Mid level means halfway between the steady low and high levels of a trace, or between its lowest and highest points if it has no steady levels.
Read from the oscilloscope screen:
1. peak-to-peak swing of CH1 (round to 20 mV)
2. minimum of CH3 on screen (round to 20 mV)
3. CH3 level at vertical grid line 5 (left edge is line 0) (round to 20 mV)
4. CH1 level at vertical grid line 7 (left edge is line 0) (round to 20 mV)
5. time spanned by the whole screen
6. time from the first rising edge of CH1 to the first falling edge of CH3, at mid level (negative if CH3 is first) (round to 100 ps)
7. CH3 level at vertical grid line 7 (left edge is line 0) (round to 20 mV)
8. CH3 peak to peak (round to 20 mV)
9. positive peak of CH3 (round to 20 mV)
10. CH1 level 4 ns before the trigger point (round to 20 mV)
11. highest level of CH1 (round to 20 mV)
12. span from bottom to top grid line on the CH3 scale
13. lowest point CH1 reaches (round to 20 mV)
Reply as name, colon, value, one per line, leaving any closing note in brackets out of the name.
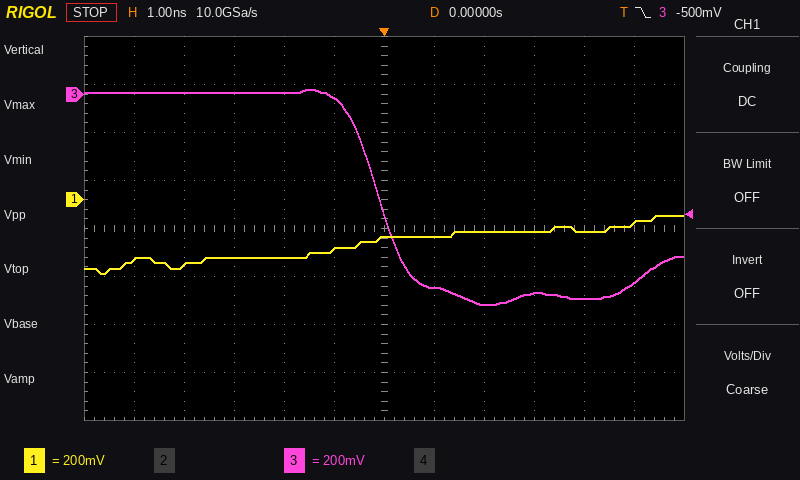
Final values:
peak-to-peak swing of CH1: 240 mV
minimum of CH3 on screen: -880 mV
CH3 level at vertical grid line 5 (left edge is line 0): -20 mV
CH1 level at vertical grid line 7 (left edge is line 0): -160 mV
time spanned by the whole screen: 12 ns
time from the first rising edge of CH1 to the first falling edge of CH3, at mid level (negative if CH3 is first): +400 ps
CH3 level at vertical grid line 7 (left edge is line 0): -800 mV
CH3 peak to peak: 900 mV
positive peak of CH3: 20 mV
CH1 level 4 ns before the trigger point: -280 mV
highest level of CH1: -60 mV
span from bottom to top grid line on the CH3 scale: 1.6 V
lowest point CH1 reaches: -300 mV
